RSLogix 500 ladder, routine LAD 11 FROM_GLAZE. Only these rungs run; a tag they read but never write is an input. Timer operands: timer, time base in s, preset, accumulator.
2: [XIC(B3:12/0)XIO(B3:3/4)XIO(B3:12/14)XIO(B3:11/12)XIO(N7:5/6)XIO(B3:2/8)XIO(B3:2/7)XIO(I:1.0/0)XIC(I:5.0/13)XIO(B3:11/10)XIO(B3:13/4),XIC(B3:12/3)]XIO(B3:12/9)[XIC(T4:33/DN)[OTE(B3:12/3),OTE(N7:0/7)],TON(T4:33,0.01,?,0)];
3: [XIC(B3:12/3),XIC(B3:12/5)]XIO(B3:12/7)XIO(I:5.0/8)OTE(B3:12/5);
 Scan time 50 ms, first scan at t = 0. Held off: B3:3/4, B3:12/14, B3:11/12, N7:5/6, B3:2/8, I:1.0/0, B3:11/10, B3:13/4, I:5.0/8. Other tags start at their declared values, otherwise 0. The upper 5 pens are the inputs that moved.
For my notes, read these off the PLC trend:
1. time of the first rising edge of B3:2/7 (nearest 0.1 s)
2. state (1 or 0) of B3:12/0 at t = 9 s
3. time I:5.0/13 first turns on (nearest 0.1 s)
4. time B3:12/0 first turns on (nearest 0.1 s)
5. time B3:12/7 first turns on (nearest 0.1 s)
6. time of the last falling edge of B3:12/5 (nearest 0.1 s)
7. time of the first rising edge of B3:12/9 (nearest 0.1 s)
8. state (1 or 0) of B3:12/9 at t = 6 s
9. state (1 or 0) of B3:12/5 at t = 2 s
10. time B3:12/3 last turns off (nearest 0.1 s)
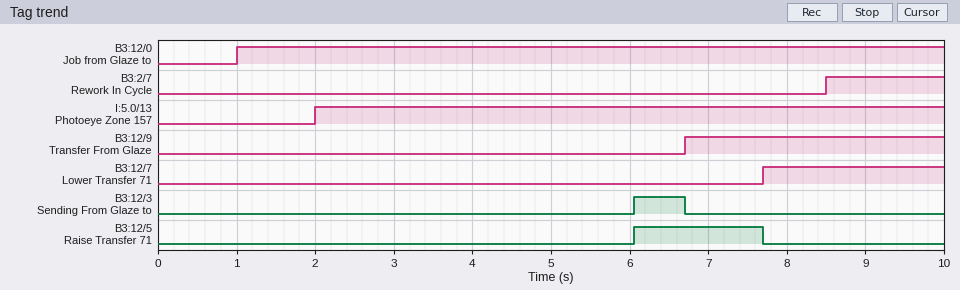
8.5 s
1
2.0 s
1.0 s
7.7 s
7.7 s
6.7 s
0
0
6.7 s
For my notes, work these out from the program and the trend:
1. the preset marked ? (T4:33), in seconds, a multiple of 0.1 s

4.0 s
